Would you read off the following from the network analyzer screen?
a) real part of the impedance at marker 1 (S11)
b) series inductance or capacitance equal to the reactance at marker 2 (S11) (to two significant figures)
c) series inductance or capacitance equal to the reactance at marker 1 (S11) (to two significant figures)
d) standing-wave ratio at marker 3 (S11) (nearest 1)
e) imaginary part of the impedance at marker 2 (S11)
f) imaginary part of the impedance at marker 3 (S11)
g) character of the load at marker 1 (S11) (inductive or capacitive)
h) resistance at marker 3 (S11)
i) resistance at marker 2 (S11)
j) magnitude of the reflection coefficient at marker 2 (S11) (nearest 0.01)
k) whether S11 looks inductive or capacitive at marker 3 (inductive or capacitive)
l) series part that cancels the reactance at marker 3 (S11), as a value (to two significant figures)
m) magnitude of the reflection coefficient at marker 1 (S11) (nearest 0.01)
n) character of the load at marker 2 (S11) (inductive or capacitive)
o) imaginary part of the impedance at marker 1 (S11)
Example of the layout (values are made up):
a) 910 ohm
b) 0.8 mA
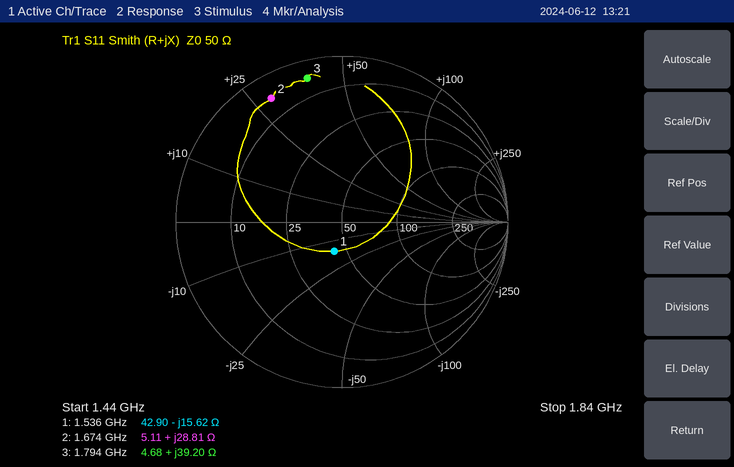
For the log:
a) 42.90 Ω
b) 2.7 nH
c) 6.6 pF
d) 17
e) +28.81 Ω
f) +39.20 Ω
g) capacitive
h) 4.68 Ω
i) 5.11 Ω
j) 0.86
k) inductive
l) 2.3 pF
m) 0.18
n) inductive
o) -15.62 Ω
